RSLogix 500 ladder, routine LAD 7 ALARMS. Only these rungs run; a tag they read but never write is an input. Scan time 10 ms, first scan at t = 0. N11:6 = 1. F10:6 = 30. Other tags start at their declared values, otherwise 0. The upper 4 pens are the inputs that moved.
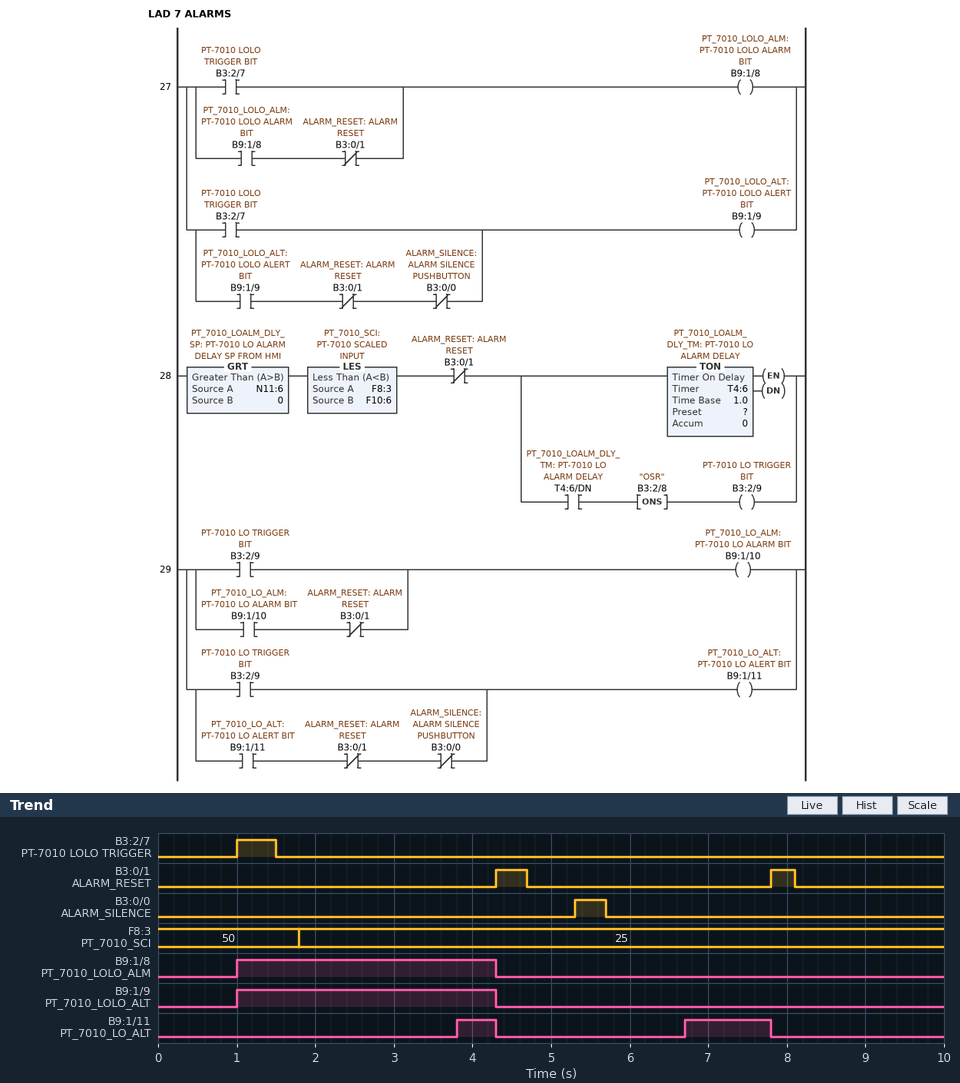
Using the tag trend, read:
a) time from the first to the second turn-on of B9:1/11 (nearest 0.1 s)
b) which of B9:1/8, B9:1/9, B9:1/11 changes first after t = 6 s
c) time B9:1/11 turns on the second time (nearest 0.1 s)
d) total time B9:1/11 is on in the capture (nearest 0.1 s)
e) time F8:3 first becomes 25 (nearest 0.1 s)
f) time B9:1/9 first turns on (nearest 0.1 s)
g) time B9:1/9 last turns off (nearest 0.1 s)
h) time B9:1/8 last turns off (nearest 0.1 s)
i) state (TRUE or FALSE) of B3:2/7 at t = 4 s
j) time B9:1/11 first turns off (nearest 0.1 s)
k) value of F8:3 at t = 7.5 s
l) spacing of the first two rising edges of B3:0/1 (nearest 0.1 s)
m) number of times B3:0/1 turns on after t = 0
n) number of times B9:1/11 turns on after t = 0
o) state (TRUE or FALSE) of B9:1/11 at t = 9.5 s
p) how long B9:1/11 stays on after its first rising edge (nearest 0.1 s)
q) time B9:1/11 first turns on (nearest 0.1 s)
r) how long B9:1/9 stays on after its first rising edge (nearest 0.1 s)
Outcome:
2.9 s
B9:1/11
6.7 s
1.6 s
1.8 s
1.0 s
4.3 s
4.3 s
FALSE
4.3 s
25
3.5 s
2
2
FALSE
0.5 s
3.8 s
3.3 s
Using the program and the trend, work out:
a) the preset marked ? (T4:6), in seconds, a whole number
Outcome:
2 s
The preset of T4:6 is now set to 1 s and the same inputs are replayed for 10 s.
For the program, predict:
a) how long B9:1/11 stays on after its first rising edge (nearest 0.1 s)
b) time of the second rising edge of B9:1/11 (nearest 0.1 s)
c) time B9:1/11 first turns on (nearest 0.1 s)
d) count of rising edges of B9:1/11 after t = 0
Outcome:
1.5 s
5.7 s
2.8 s
3
